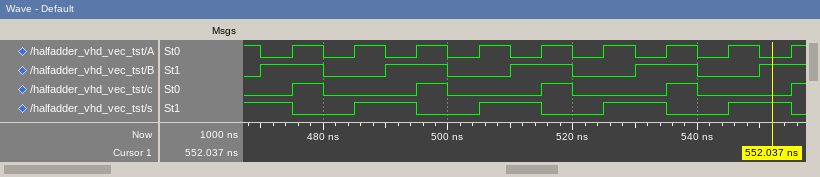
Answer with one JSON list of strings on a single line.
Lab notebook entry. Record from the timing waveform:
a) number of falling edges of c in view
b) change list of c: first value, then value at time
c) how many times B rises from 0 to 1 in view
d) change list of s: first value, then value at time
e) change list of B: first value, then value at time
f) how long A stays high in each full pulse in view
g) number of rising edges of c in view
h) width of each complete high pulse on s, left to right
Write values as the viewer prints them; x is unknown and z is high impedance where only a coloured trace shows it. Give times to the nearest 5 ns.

["4", "0, 1 at 475 ns, 0 at 480 ns, 1 at 495 ns, 0 at 500 ns, 1 at 515 ns, 0 at 520 ns, 1 at 535 ns, 0 at 540 ns, 1 at 555 ns", "5", "1, 0 at 475 ns, 1 at 485 ns, 0 at 495 ns, 1 at 505 ns, 0 at 515 ns, 1 at 525 ns, 0 at 535 ns, 1 at 545 ns, 0 at 555 ns", "0, 1 at 470 ns, 0 at 480 ns, 1 at 490 ns, 0 at 500 ns, 1 at 510 ns, 0 at 520 ns, 1 at 530 ns, 0 at 540 ns, 1 at 550 ns", "5 ns, 5 ns, 5 ns, 5 ns, 5 ns, 5 ns, 5 ns, 5 ns", "5", "10 ns, 10 ns, 10 ns, 10 ns"]
